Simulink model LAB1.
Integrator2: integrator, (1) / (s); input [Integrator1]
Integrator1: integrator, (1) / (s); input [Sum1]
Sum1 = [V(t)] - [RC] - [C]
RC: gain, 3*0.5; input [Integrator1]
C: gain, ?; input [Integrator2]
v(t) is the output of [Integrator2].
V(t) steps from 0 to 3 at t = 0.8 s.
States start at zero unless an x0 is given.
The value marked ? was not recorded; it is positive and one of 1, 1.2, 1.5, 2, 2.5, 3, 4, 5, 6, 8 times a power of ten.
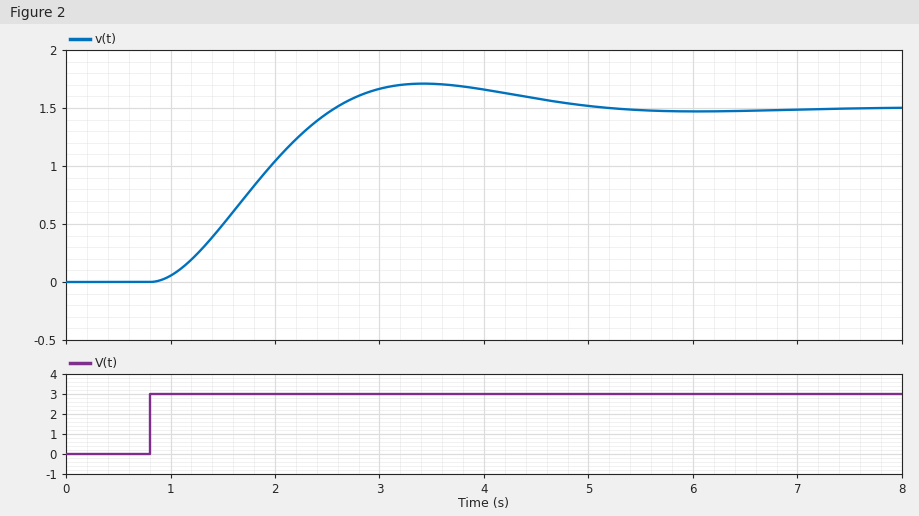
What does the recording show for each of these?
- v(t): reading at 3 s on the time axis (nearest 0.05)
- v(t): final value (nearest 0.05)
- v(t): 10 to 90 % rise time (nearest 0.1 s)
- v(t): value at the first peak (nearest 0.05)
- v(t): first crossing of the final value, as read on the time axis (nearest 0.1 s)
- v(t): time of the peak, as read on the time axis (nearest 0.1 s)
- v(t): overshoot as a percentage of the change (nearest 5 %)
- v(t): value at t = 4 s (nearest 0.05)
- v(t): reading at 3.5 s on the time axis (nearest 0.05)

1.65
1.50
1.2 s
1.70
2.6 s
3.4 s
15 %
1.65
1.70
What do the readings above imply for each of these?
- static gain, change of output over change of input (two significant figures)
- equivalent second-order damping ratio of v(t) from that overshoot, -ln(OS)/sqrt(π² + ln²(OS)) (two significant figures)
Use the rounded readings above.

0.50
0.52
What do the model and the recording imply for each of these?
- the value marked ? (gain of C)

2
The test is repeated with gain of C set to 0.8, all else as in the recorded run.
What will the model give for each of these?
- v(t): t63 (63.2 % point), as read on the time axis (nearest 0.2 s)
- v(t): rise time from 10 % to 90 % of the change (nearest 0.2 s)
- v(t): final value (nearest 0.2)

3.0 s
3.0 s
3.8
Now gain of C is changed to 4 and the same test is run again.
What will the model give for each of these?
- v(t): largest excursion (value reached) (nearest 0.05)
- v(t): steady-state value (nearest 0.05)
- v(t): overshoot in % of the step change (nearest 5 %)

0.95
0.75
30 %
